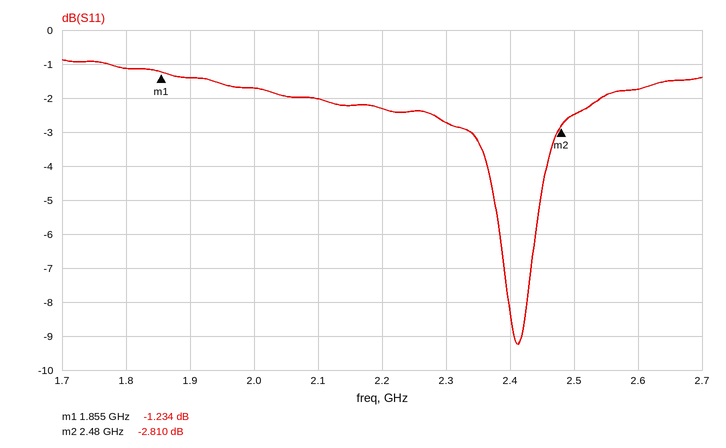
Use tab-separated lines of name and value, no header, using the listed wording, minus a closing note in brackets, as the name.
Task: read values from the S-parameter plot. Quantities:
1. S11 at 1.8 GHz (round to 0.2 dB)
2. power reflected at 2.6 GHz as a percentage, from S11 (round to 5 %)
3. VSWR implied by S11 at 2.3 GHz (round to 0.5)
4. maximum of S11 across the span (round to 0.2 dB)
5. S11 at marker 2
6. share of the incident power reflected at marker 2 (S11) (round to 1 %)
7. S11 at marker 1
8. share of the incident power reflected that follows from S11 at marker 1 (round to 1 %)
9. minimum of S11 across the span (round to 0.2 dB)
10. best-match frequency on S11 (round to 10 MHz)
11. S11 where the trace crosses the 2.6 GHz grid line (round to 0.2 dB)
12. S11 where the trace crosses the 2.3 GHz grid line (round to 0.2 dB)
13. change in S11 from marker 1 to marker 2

S11 at 1.8 GHz	-1.2 dB
power reflected at 2.6 GHz as a percentage, from S11	65 %
VSWR implied by S11 at 2.3 GHz	6.5
maximum of S11 across the span	-0.8 dB
S11 at marker 2	-2.810 dB
share of the incident power reflected at marker 2 (S11)	52 %
S11 at marker 1	-1.234 dB
share of the incident power reflected that follows from S11 at marker 1	75 %
minimum of S11 across the span	-9.2 dB
best-match frequency on S11	2.41 GHz
S11 where the trace crosses the 2.6 GHz grid line	-1.8 dB
S11 where the trace crosses the 2.3 GHz grid line	-2.8 dB
change in S11 from marker 1 to marker 2	-1.576 dB
